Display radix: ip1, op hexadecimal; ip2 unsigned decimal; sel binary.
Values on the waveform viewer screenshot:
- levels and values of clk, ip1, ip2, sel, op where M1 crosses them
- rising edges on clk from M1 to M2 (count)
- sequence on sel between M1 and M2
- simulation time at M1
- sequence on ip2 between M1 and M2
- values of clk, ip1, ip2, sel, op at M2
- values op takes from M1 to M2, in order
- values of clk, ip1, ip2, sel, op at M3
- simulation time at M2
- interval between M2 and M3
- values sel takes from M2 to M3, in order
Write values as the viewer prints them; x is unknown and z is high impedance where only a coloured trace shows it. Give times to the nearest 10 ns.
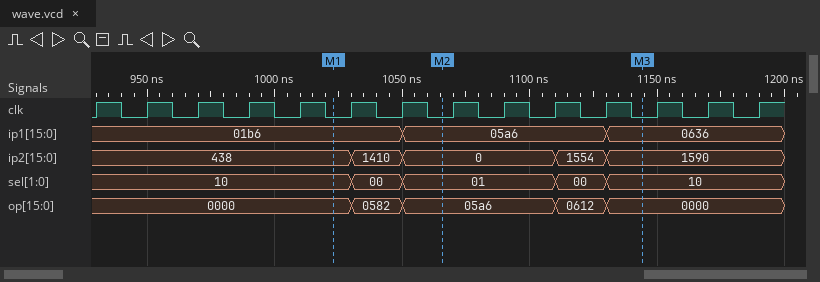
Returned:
clk=0, ip1=01b6, ip2=438, sel=10, op=0000
2
10, 00, 01
1020 ns
438, 1410, 0
clk=0, ip1=05a6, ip2=0, sel=01, op=05a6
0000, 0582, 05a6
clk=0, ip1=0636, ip2=1590, sel=10, op=0000
1070 ns
80 ns
01, 00, 10
